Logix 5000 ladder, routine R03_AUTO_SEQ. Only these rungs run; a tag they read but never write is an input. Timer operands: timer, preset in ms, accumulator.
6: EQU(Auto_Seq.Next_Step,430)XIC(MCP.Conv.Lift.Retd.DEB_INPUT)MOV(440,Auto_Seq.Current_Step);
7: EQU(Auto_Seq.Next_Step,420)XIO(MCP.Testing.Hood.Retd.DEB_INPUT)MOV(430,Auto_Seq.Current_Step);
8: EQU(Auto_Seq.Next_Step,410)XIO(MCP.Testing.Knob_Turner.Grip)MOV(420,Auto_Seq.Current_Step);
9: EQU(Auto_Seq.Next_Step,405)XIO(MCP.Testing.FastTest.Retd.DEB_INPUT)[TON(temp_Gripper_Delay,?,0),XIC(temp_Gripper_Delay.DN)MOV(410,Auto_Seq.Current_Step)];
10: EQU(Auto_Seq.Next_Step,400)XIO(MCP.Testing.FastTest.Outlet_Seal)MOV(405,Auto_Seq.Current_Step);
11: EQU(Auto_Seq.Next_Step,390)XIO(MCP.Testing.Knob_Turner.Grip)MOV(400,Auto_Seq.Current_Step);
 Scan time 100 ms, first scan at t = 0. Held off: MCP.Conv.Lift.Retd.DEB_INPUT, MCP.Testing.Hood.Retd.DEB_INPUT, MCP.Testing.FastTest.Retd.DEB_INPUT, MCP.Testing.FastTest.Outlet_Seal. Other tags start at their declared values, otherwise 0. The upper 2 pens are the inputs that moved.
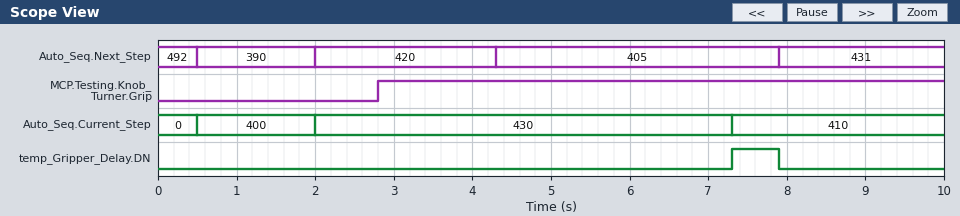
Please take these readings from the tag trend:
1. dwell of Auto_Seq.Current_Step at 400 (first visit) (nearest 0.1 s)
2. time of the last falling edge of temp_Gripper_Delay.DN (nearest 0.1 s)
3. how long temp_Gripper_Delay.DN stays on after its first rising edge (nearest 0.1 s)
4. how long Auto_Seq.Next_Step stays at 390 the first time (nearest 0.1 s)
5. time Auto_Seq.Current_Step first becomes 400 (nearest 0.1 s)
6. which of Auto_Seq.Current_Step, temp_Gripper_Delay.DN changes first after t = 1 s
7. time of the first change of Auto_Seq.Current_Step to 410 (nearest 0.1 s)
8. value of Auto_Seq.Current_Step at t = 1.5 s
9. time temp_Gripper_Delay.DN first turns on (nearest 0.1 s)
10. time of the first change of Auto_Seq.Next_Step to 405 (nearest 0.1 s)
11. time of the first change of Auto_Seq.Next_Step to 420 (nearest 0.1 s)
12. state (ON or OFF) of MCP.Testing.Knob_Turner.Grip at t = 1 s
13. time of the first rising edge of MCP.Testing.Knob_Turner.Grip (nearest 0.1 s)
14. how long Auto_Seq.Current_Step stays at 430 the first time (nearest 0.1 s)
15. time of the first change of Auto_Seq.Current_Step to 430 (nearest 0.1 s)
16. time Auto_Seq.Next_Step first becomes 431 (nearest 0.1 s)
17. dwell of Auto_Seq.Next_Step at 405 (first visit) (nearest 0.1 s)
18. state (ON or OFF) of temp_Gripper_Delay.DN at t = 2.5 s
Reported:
1.5 s
7.9 s
0.6 s
1.5 s
0.5 s
Auto_Seq.Current_Step
7.3 s
400
7.3 s
4.3 s
2.0 s
OFF
2.8 s
5.3 s
2.0 s
7.9 s
3.6 s
OFF
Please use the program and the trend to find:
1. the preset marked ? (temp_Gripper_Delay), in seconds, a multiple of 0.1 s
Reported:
3.0 s
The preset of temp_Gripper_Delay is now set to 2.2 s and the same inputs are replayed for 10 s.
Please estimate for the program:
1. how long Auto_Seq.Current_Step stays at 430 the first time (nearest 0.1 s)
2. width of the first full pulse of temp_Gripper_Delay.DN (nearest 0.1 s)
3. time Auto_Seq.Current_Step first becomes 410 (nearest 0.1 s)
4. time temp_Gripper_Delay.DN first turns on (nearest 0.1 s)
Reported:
4.5 s
1.4 s
6.5 s
6.5 s
